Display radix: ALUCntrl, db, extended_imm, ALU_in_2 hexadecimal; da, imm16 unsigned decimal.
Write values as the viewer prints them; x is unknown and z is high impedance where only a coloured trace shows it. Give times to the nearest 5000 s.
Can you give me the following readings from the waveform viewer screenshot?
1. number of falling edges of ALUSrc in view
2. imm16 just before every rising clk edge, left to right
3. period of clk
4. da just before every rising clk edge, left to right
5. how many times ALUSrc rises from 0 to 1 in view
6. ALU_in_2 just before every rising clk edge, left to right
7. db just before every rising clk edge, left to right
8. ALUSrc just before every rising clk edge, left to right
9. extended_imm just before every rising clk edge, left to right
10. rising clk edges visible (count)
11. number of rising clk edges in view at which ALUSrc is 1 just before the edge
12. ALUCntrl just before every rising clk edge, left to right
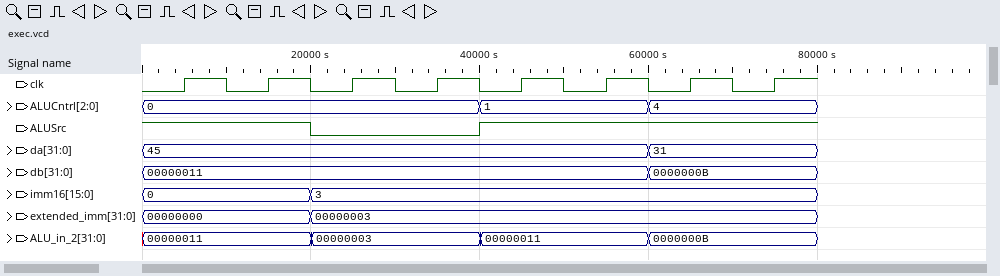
1
0, 0, 3, 3, 3, 3, 3, 3
10000 s
45, 45, 45, 45, 45, 45, 31, 31
1
00000011, 00000011, 00000003, 00000003, 00000011, 00000011, 0000000B, 0000000B
00000011, 00000011, 00000011, 00000011, 00000011, 00000011, 0000000B, 0000000B
1 1 0 0 1 1 1 1
00000000, 00000000, 00000003, 00000003, 00000003, 00000003, 00000003, 00000003
8
6
0, 0, 0, 0, 1, 1, 4, 4
